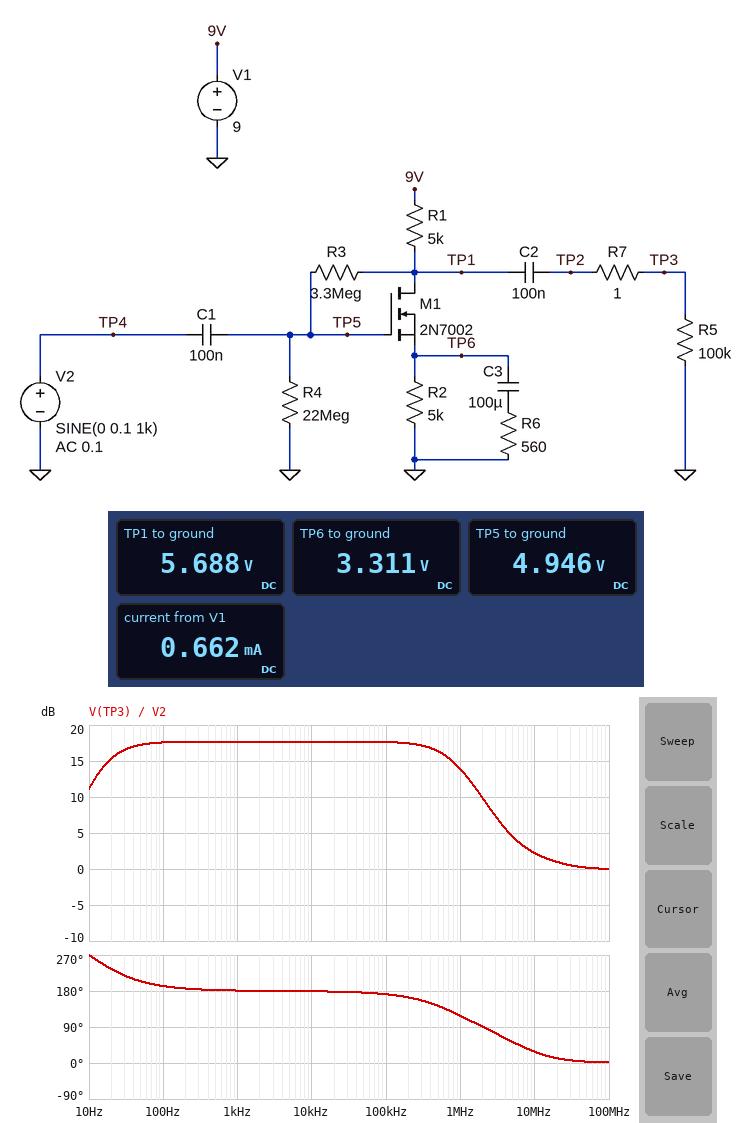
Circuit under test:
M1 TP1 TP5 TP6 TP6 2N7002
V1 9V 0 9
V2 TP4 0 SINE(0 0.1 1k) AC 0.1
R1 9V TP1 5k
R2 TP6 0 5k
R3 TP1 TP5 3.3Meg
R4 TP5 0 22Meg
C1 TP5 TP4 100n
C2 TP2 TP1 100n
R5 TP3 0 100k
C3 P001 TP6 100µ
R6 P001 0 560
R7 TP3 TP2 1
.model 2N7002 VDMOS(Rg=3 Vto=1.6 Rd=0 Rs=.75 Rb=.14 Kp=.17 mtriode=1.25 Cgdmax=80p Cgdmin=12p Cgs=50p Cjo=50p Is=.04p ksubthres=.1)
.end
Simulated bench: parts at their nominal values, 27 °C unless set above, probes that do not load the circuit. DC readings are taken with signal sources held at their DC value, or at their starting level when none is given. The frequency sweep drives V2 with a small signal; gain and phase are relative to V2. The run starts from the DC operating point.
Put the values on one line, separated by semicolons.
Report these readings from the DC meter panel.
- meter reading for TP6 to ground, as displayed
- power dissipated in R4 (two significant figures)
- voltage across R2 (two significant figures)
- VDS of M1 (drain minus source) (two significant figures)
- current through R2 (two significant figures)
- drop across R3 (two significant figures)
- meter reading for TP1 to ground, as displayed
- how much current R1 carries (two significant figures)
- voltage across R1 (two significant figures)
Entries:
3.311 V; 1.1 µW; 3.3 V; 2.4 V; 660 µA; 740 mV; 5.688 V; 660 µA; 3.3 V
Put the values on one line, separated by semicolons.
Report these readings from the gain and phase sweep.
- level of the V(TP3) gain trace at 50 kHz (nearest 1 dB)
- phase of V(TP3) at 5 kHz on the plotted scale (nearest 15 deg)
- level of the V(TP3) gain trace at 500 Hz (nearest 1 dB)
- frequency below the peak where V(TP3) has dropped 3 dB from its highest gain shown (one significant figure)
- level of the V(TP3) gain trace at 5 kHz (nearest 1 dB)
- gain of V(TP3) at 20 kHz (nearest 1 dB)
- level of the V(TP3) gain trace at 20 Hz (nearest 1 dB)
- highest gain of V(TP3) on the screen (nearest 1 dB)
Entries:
18 dB; 180 deg; 18 dB; 20 Hz; 18 dB; 18 dB; 15 dB; 18 dB
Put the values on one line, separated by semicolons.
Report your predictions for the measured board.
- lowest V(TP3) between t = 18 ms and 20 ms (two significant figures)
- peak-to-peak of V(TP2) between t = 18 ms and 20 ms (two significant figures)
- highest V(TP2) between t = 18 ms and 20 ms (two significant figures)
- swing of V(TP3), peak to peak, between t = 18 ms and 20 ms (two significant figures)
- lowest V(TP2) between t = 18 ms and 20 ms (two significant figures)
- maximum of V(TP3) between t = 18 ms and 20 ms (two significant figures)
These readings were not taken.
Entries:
-770 mV; 1.5 V; 760 mV; 1.5 V; -770 mV; 760 mV
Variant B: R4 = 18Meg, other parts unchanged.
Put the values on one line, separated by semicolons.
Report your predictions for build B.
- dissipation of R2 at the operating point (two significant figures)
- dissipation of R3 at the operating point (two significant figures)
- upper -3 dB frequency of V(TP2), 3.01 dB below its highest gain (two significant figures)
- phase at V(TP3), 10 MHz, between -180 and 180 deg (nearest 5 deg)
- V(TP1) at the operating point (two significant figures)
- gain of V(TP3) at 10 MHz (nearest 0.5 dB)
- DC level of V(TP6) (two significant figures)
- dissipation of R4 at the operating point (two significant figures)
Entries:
2.1 mW; 240 nW; 890 kHz; 30 deg; 5.8 V; 2.5 dB; 3.2 V; 1.3 µW
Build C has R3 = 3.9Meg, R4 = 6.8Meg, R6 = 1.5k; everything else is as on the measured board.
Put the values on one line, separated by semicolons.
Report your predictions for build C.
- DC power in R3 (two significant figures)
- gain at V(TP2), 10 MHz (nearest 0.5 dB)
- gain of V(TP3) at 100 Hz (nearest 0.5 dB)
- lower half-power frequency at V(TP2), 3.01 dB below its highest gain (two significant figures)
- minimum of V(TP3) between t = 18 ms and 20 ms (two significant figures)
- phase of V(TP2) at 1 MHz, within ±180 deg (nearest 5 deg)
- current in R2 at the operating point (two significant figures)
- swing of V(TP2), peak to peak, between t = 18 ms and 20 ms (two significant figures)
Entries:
1.4 µW; 2.0 dB; 11.0 dB; 16 Hz; -370 mV; 130 deg; 500 µA; 730 mV
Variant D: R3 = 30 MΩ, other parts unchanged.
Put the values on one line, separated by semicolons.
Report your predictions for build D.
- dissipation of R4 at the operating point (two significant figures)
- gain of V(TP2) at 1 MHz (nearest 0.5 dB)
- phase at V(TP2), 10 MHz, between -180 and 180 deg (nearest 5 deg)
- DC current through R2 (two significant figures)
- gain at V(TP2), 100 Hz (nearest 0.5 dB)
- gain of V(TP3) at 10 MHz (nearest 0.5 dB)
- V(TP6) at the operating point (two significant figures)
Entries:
450 nW; 15.0 dB; 35 deg; 310 µA; 16.5 dB; 3.5 dB; 1.6 V
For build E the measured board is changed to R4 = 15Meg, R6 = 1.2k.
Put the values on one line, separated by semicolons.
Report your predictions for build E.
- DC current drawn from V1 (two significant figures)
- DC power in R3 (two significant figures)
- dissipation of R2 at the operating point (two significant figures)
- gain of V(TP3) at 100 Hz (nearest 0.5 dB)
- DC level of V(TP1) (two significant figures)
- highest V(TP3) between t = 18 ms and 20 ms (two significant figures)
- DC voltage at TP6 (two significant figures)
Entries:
630 µA; 340 nW; 2.0 mW; 12.5 dB; 5.8 V; 440 mV; 3.2 V
